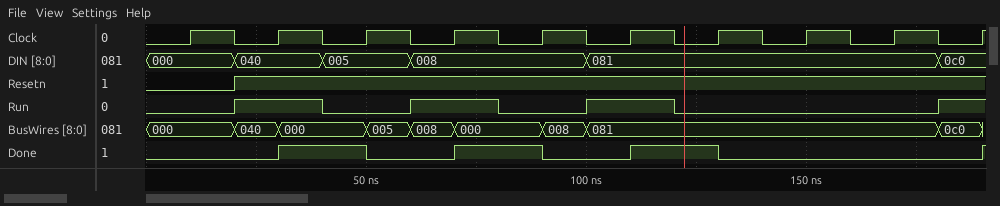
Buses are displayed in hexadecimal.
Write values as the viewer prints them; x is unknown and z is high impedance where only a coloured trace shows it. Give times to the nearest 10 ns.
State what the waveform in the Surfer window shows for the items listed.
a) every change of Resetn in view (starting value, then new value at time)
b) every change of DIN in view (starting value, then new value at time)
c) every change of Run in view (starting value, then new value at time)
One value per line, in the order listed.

0, 1 at 20 ns
000, 040 at 20 ns, 005 at 40 ns, 008 at 60 ns, 081 at 100 ns, 0c0 at 180 ns
0, 1 at 20 ns, 0 at 40 ns, 1 at 60 ns, 0 at 80 ns, 1 at 100 ns, 0 at 120 ns, 1 at 180 ns
